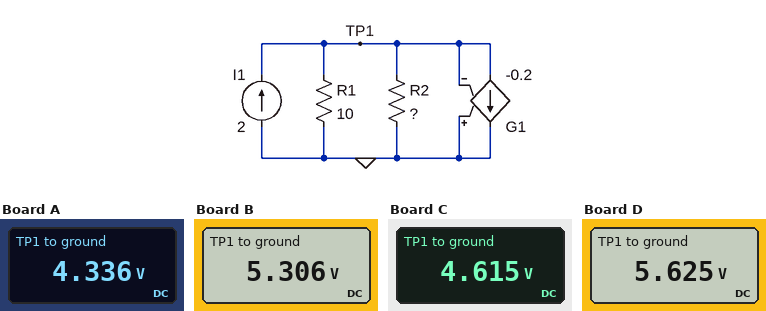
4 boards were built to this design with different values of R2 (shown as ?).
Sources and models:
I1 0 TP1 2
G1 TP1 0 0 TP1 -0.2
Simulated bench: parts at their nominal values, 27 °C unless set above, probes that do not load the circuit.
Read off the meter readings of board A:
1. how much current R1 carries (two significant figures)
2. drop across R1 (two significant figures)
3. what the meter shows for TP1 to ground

430 mA
4.3 V
4.336 V
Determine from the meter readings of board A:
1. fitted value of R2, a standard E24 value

6.2 Ω
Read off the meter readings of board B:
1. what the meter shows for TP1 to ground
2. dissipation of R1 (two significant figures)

5.306 V
2.8 W
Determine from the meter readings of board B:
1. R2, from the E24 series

13 Ω
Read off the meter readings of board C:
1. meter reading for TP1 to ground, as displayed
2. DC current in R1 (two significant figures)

4.615 V
460 mA
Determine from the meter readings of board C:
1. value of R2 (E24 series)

7.5 Ω
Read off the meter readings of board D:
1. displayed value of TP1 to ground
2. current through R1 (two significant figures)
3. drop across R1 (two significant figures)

5.625 V
560 mA
5.6 V
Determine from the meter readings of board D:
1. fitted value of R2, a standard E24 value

18 Ω
